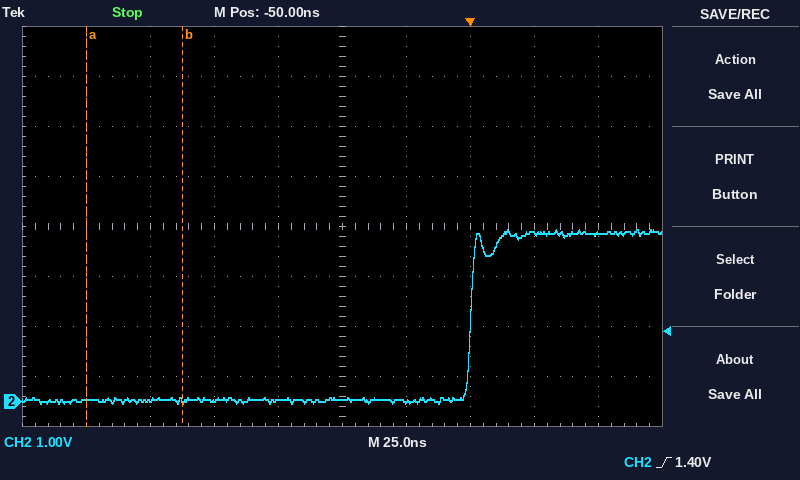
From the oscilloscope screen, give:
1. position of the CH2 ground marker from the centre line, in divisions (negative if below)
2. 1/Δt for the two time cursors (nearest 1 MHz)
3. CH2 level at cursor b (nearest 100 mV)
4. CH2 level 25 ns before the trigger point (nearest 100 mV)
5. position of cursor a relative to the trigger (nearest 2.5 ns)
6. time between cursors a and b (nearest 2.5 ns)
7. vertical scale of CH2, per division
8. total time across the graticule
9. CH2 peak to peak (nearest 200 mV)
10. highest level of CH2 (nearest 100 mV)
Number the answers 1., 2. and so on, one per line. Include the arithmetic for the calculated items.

1. -3.5 div
2. 1 / 37.5 ns ≈ 27 MHz
3. 0.0 V
4. 0.0 V
5. -150.0 ns
6. 37.5 ns
7. 1 V
8. 250 ns
9. 3.4 V
10. 3.4 V
